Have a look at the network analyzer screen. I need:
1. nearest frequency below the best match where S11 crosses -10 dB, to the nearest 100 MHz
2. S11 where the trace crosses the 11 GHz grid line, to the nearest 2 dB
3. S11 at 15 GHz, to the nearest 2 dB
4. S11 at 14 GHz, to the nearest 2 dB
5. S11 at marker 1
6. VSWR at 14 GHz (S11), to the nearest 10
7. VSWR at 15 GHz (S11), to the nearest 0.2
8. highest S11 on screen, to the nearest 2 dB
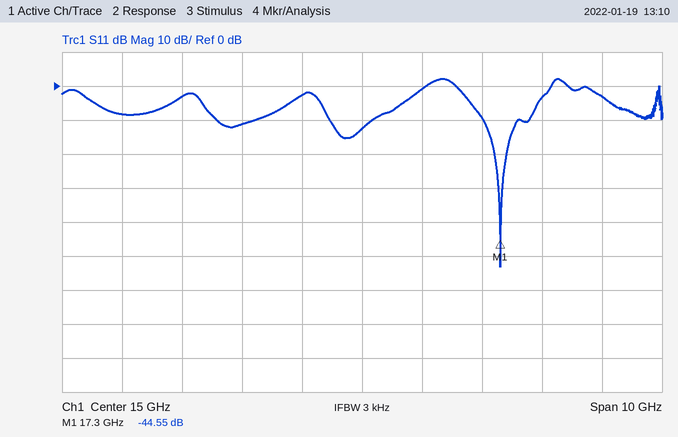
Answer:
17.0 GHz
-8 dB
-12 dB
-2 dB
-44.55 dB
10
1.6
2 dB
